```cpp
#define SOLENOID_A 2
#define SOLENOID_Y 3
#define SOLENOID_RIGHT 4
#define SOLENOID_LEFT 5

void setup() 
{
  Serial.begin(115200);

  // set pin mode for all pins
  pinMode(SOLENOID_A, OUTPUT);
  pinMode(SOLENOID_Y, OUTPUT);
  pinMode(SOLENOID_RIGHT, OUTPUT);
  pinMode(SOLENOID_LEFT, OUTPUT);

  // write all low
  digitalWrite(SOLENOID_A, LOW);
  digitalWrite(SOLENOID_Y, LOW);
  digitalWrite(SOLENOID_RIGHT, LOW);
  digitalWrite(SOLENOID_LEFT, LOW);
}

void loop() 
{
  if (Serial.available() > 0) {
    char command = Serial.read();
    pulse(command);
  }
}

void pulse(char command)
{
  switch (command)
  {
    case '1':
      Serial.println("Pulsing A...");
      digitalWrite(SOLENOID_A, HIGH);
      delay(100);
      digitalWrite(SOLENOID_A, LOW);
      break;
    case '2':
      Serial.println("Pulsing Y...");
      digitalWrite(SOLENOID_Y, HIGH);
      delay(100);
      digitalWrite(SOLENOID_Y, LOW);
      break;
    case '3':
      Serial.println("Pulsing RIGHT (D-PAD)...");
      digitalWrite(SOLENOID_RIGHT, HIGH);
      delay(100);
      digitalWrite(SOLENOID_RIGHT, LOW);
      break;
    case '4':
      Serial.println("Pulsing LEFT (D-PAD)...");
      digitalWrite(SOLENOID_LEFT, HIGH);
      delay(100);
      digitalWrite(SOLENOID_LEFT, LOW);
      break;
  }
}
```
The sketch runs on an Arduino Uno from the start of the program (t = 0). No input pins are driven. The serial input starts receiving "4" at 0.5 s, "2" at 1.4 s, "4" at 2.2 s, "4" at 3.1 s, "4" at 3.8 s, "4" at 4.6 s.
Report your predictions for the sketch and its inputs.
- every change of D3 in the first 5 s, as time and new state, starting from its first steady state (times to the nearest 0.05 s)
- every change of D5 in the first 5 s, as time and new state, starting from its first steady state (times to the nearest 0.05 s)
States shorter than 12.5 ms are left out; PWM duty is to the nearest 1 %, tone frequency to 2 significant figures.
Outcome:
0 s low; 1.4 s high; 1.5 s low
0 s low; 0.5 s high; 0.6 s low; 2.2 s high; 2.3 s low; 3.1 s high; 3.2 s low; 3.8 s high; 3.9 s low; 4.6 s high; 4.7 s low
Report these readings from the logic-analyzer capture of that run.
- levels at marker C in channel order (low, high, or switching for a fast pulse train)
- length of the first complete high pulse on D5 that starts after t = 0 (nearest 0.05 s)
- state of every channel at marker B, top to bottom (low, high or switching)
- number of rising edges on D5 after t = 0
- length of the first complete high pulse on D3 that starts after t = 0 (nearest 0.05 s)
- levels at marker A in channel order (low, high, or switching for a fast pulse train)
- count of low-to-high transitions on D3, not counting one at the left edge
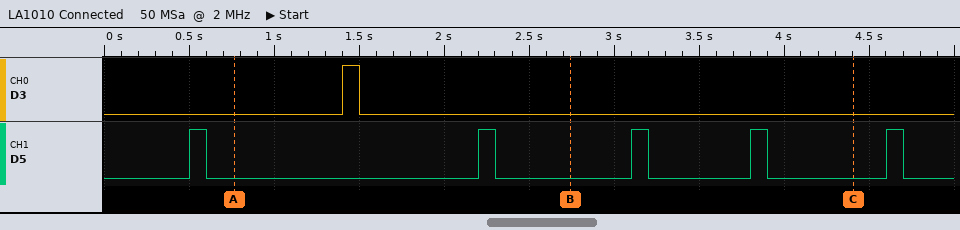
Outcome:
D3 low, D5 low
0.10 s
D3 low, D5 low
5
0.10 s
D3 low, D5 low
1
